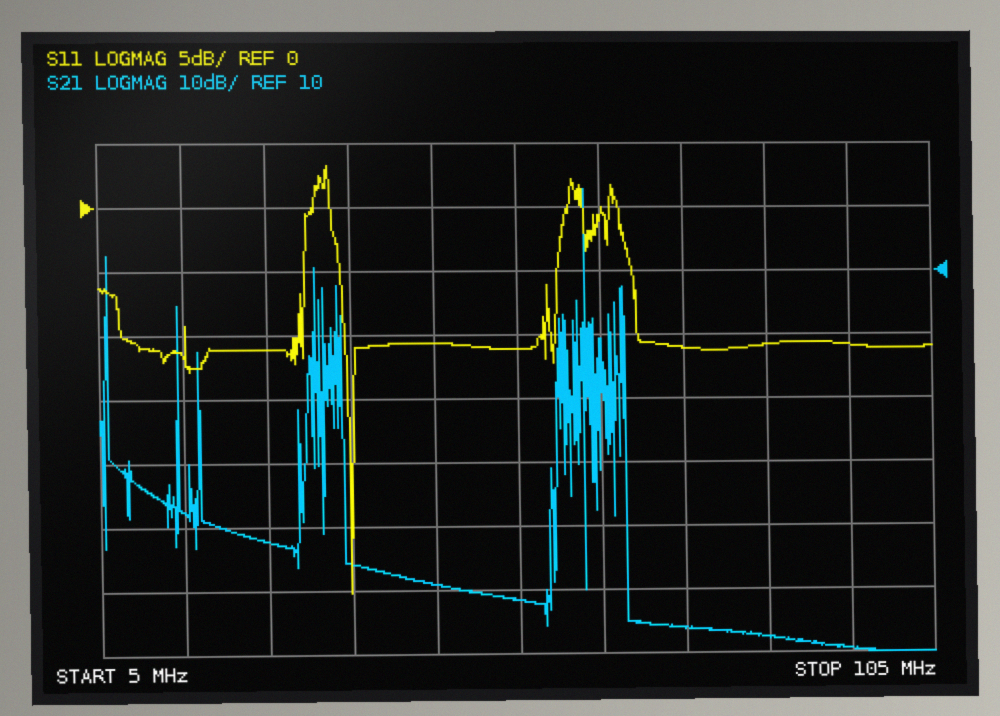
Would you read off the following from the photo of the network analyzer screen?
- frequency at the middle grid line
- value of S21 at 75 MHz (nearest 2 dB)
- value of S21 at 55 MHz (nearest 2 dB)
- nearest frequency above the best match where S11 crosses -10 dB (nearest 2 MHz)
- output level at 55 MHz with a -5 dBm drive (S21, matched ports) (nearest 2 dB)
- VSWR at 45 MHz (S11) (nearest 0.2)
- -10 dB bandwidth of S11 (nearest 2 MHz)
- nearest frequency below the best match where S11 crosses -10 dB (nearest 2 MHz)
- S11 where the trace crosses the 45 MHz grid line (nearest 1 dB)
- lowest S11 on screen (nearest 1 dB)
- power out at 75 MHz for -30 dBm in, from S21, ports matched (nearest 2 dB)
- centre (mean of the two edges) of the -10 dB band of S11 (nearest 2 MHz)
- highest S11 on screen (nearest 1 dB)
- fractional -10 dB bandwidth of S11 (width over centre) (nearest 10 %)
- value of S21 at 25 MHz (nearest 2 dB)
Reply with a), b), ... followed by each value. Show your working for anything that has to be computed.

a) 55 MHz
b) -46 dB
c) -42 dB
d) 58 MHz
e) -5 dBm + (-42 dB) = -46 dBm
f) |Γ| = 10^(-11/20) = 0.2818; VSWR = (1 + 0.2818)/(1 − 0.2818) ≈ 1.8
g) 58 MHz − 34 MHz = 24 MHz
h) 34 MHz
i) -11 dB
j) -30 dB
k) -30 dBm + (-46 dB) = -76 dBm
l) 46 MHz
m) 3 dB
n) 24 MHz / 46 MHz ≈ 52.2 %, so 50 % to the nearest 10 %
o) -32 dB
